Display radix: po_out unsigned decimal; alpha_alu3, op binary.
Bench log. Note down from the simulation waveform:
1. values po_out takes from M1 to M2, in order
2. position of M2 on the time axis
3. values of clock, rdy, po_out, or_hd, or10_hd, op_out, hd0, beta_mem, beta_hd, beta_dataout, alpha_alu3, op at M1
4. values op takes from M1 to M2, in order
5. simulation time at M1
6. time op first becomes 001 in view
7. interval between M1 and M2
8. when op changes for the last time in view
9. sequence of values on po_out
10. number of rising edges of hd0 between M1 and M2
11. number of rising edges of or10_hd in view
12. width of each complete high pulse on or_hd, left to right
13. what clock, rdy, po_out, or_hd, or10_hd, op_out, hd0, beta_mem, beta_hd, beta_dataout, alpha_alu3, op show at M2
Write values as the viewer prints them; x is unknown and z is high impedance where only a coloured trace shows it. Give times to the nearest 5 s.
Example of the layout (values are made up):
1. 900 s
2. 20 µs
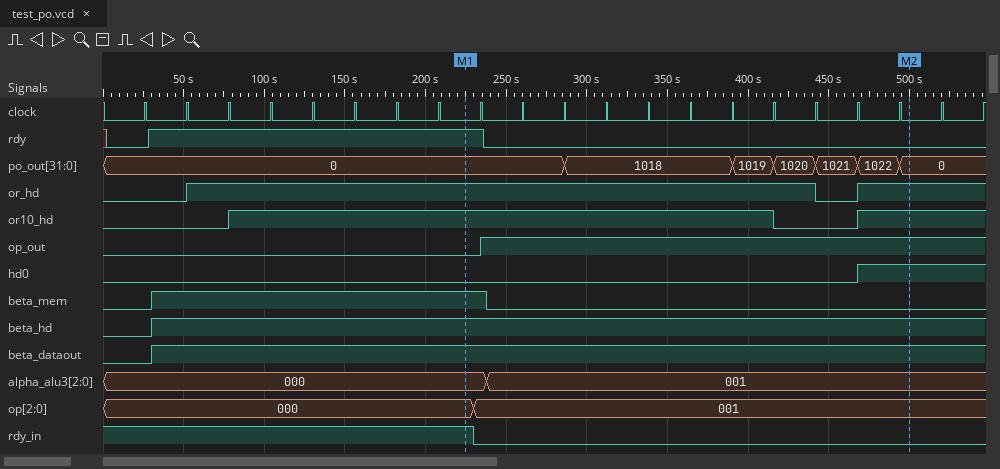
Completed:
1. 0, 1018, 1019, 1020, 1021, 1022, 0
2. 500 s
3. clock=0, rdy=1, po_out=0, or_hd=1, or10_hd=1, op_out=0, hd0=0, beta_mem=1, beta_hd=1, beta_dataout=1, alpha_alu3=000, op=000
4. 000, 001
5. 225 s
6. 230 s
7. 275 s
8. 230 s
9. 0, 1018, 1019, 1020, 1021, 1022, 0
10. 1
11. 2
12. 390 s
13. clock=0, rdy=0, po_out=0, or_hd=1, or10_hd=1, op_out=1, hd0=1, beta_mem=0, beta_hd=1, beta_dataout=1, alpha_alu3=001, op=001
